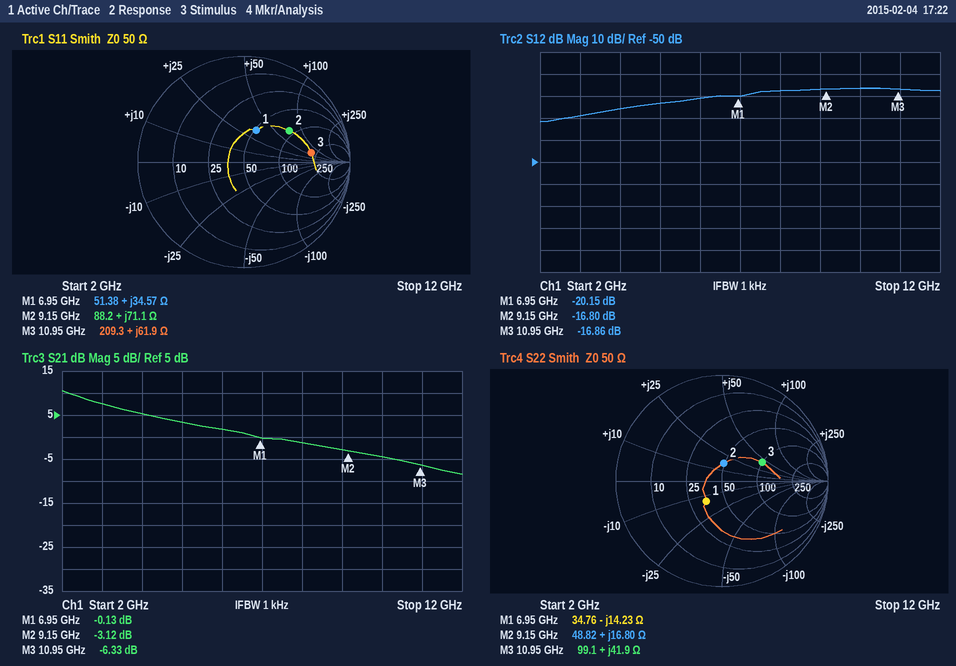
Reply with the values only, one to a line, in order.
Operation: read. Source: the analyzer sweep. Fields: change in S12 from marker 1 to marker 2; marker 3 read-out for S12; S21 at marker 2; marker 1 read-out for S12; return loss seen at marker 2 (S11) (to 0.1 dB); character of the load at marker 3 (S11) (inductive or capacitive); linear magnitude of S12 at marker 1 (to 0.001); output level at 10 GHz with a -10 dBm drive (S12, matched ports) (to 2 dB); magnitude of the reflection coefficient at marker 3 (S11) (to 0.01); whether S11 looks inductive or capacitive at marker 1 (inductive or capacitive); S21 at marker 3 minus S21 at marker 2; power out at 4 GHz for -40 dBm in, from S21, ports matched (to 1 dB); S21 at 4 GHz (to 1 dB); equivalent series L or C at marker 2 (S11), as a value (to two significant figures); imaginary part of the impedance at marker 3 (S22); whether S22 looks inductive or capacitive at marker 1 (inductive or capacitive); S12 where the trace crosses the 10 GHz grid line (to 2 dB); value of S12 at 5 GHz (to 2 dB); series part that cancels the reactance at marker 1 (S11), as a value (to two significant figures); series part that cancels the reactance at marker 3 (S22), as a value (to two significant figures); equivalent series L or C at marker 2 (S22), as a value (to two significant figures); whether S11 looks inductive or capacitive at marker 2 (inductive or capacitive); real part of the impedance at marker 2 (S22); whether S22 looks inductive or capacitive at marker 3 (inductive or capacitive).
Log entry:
3.35 dB
-16.86 dB
-3.12 dB
-20.15 dB
5.7 dB
inductive
0.098
-26 dBm
0.64
inductive
-3.21 dB
-35 dBm
5 dB
1.2 nH
+41.9 Ω
capacitive
-16 dB
-24 dB
660 fF
350 fF
290 pH
inductive
48.82 Ω
inductive
